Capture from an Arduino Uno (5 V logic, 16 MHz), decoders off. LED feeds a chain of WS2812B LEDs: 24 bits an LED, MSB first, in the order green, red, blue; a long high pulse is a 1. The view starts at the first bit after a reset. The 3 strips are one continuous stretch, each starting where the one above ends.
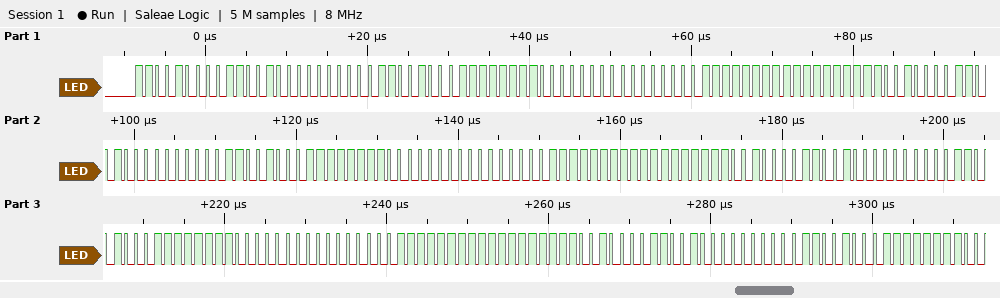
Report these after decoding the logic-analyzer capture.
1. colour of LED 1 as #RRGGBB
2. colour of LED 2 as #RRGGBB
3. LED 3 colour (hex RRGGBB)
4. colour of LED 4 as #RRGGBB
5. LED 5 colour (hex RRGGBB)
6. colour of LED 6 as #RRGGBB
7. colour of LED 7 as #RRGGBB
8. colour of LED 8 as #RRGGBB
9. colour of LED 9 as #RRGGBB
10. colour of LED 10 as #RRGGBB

#64C800
#FFC800
#FF00FF
#64C800
#FFC800
#FF00FF
#64C800
#FFC800
#FF00FF
#64C800
